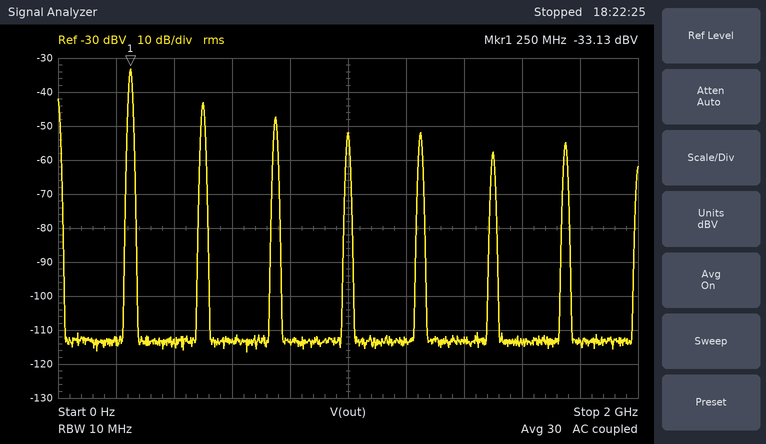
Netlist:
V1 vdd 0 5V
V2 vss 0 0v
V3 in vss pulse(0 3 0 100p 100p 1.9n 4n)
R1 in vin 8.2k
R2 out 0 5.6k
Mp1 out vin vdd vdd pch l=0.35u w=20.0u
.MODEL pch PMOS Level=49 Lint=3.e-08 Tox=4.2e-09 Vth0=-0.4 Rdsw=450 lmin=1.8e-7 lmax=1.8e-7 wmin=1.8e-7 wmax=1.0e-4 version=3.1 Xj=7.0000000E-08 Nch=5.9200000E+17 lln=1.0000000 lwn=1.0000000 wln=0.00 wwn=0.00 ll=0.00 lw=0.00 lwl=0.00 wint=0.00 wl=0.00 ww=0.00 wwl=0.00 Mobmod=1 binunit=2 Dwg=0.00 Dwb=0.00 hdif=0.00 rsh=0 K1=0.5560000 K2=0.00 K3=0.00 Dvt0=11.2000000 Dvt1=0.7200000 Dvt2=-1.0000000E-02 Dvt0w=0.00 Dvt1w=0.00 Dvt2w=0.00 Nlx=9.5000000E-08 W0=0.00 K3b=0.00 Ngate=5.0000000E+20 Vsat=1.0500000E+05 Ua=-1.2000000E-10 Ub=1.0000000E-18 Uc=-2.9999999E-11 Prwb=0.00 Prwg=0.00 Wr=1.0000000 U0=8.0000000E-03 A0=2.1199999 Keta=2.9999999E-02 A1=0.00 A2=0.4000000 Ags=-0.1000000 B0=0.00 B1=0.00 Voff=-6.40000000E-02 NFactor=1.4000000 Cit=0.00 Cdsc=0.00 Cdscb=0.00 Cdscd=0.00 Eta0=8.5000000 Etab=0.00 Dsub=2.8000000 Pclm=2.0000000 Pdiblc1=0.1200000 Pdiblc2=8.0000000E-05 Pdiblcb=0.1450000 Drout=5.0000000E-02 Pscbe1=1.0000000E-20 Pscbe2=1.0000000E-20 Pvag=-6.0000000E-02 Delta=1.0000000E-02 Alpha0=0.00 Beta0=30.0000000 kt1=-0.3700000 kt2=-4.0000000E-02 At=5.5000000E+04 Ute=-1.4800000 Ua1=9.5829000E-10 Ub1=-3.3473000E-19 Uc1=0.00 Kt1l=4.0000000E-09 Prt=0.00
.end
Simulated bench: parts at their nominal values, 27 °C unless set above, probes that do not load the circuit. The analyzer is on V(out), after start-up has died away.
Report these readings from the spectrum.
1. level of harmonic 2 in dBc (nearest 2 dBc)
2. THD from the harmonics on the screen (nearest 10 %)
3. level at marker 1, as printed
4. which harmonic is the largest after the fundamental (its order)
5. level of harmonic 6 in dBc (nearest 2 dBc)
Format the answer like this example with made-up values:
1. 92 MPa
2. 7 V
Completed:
1. -10 dBc
2. 40 %
3. -33.13 dBV
4. 2
5. -24 dBc
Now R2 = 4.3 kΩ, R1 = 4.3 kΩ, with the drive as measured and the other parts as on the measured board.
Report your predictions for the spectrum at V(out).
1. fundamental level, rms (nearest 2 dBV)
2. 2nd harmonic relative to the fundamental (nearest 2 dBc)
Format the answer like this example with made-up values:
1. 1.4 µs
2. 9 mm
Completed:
1. -28 dBV
2. -12 dBc
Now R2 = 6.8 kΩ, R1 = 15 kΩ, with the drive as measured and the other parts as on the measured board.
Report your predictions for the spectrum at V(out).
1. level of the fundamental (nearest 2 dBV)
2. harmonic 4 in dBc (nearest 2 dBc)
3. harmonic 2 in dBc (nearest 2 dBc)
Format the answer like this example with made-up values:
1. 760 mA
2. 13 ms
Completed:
1. -38 dBV
2. -22 dBc
3. -12 dBc
